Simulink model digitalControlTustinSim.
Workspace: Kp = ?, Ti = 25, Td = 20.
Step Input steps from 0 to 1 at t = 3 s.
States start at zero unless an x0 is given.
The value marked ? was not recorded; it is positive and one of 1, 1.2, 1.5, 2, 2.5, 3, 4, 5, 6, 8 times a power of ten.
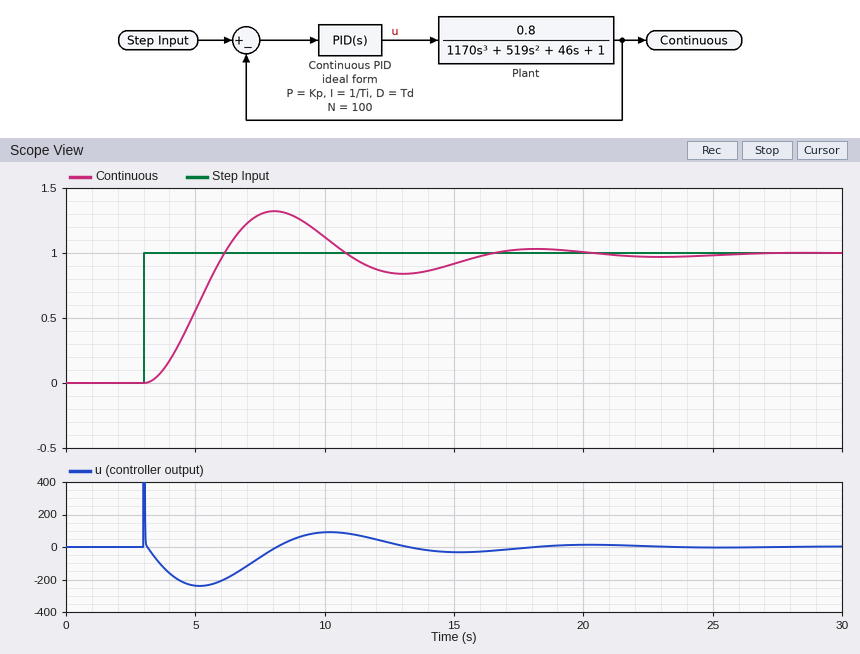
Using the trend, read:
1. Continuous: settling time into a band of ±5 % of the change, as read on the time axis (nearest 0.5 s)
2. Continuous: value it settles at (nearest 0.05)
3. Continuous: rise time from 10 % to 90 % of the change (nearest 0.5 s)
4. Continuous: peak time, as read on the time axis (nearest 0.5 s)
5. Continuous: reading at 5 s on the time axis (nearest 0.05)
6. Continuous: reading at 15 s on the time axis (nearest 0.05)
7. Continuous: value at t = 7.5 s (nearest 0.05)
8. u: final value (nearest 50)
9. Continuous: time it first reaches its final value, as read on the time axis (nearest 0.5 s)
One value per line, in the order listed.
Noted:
15.5 s
1.00
2.0 s
8.0 s
0.55
0.90
1.30
0
6.0 s
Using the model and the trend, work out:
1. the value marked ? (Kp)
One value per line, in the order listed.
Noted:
30
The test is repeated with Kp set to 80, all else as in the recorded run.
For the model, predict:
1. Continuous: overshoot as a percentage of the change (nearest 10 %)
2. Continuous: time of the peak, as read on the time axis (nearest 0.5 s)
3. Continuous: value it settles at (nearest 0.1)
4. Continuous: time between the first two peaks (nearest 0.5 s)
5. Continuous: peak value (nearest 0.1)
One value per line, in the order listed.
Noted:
50 %
6.0 s
1.0
6.0 s
1.5
